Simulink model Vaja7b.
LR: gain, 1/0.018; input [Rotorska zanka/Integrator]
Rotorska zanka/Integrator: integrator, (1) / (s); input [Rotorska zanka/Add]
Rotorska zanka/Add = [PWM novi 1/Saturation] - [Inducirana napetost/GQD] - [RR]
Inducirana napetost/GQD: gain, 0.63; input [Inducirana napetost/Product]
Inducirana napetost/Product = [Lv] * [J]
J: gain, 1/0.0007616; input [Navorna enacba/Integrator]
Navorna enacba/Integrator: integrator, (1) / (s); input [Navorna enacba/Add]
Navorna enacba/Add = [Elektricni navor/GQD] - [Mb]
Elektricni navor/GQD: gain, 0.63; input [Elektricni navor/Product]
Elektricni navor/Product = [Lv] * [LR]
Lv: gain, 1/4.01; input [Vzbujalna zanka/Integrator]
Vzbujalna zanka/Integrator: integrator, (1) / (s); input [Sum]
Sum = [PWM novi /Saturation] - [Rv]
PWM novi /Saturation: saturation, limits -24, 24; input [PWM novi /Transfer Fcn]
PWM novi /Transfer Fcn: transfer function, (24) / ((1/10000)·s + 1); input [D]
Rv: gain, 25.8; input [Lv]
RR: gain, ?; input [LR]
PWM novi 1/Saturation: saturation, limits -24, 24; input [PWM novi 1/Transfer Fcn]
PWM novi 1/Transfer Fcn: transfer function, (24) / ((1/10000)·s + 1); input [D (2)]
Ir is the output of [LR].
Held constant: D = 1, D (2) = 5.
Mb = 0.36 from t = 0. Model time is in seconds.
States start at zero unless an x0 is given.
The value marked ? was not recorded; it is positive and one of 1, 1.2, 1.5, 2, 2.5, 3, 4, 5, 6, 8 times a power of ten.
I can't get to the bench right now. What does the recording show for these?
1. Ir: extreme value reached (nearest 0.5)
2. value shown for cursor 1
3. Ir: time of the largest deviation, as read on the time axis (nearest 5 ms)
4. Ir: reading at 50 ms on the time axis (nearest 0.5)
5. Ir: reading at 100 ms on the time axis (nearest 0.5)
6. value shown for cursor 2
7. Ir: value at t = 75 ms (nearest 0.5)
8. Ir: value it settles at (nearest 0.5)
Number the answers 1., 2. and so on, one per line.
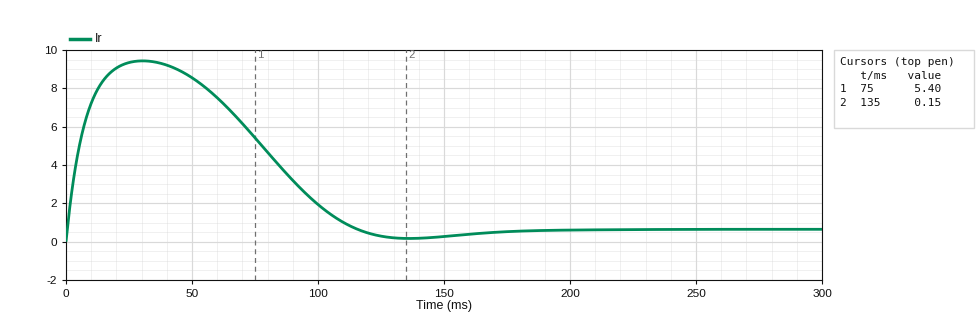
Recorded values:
1. 9.5
2. 5.40
3. 30 ms
4. 8.5
5. 2.0
6. 0.15
7. 5.5
8. 0.5
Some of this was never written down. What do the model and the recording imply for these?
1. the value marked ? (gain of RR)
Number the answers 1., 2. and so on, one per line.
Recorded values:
1. 2.5
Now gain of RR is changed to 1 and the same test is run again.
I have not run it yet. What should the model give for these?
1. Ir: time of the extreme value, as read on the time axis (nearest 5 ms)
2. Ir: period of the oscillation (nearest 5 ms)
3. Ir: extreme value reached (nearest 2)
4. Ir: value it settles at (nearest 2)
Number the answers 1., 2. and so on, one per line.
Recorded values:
1. 35 ms
2. 105 ms
3. 20
4. 0
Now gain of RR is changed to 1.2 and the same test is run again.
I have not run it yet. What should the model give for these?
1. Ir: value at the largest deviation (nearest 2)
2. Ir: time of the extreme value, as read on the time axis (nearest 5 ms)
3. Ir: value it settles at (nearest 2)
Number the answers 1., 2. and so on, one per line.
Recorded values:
1. 18
2. 35 ms
3. 0
